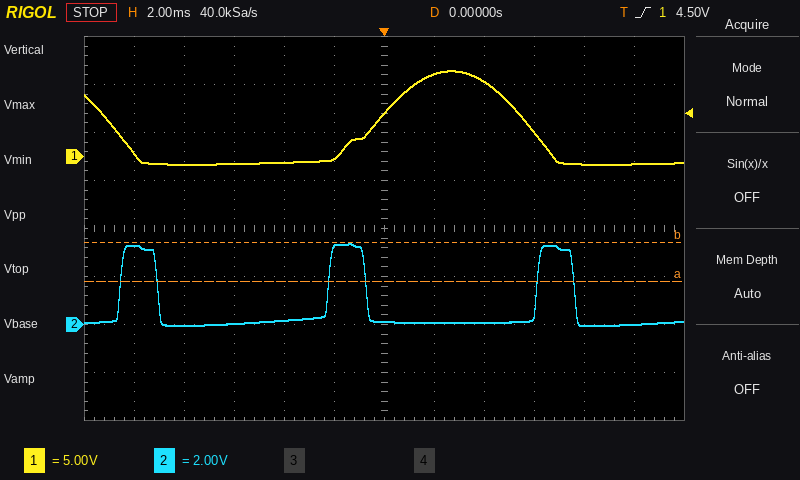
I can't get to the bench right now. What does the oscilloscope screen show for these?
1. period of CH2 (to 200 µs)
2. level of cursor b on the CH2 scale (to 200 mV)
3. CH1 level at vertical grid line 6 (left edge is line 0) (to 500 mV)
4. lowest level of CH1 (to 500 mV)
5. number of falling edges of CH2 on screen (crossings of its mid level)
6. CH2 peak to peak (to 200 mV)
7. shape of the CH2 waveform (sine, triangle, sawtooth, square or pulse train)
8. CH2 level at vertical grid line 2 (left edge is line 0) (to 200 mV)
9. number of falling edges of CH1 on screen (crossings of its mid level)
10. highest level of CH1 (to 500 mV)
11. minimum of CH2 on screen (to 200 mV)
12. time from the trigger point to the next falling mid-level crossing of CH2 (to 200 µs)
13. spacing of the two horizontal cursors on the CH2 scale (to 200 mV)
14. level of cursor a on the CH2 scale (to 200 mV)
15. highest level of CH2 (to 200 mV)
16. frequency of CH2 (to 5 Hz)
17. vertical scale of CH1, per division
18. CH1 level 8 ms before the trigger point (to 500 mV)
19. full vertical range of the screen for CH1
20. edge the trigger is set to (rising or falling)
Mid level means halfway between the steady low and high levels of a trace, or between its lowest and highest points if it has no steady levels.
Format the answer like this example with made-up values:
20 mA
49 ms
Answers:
8.4 ms
3.4 V
4.5 V
-1.0 V
3
3.4 V
pulse train
0.0 V
2
9.0 V
0.0 V
7.6 ms
1.6 V
1.8 V
3.4 V
120 Hz
5 V
-1.0 V
40 V
rising
